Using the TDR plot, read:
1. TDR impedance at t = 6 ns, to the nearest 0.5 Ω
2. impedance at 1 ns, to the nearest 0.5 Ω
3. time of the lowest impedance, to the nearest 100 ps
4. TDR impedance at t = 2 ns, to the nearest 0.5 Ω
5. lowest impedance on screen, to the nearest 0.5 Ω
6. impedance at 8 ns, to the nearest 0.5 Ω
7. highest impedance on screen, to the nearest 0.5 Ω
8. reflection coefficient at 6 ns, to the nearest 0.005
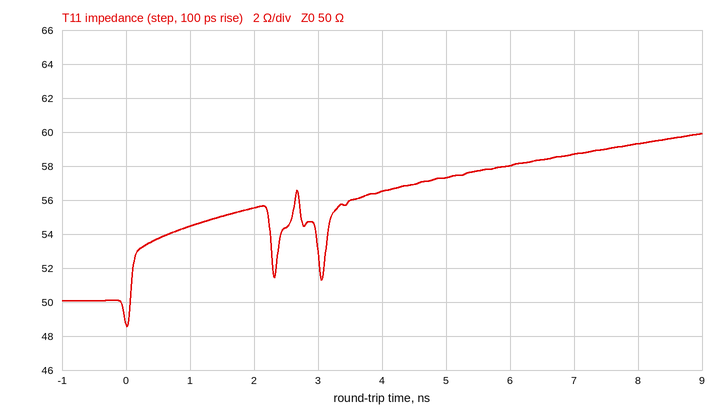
58.0 Ω
54.5 Ω
0.0 ns
55.5 Ω
48.5 Ω
59.5 Ω
60.0 Ω
+0.075
